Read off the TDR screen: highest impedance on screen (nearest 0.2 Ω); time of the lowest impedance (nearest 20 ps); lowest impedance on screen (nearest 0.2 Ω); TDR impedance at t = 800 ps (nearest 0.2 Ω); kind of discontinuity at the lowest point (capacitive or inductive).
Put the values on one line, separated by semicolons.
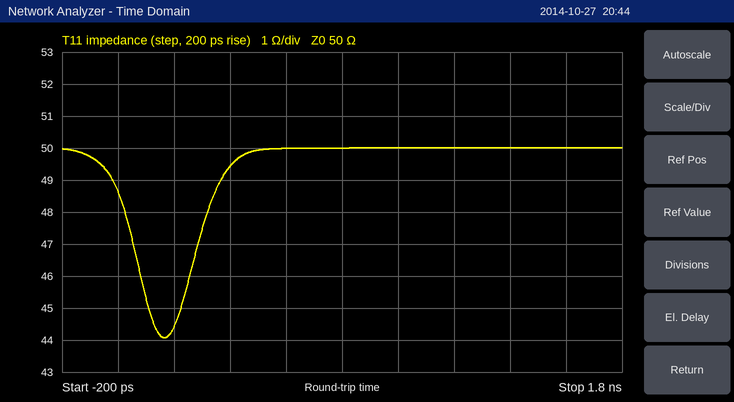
50.0 Ω; 160 ps; 44.0 Ω; 50.0 Ω; capacitive
